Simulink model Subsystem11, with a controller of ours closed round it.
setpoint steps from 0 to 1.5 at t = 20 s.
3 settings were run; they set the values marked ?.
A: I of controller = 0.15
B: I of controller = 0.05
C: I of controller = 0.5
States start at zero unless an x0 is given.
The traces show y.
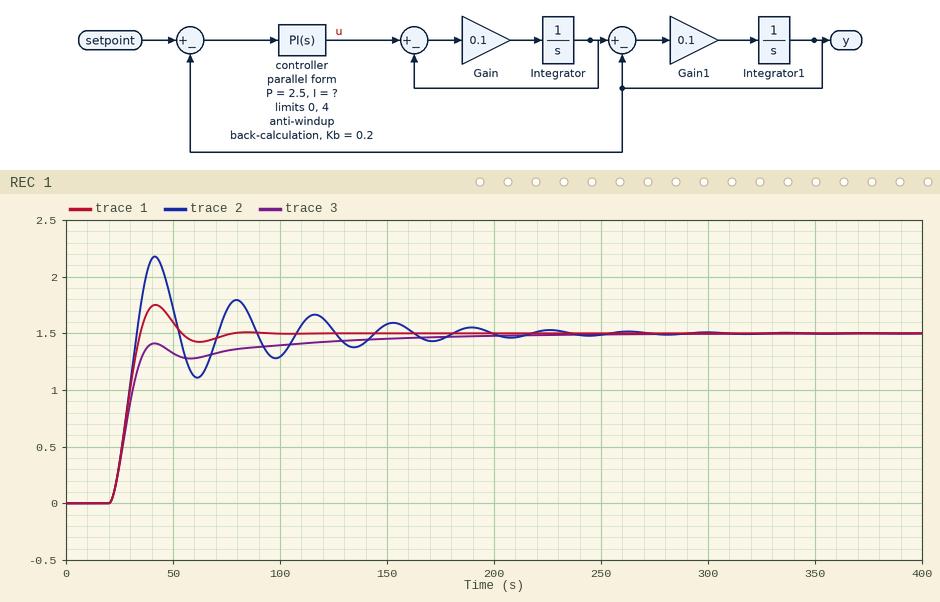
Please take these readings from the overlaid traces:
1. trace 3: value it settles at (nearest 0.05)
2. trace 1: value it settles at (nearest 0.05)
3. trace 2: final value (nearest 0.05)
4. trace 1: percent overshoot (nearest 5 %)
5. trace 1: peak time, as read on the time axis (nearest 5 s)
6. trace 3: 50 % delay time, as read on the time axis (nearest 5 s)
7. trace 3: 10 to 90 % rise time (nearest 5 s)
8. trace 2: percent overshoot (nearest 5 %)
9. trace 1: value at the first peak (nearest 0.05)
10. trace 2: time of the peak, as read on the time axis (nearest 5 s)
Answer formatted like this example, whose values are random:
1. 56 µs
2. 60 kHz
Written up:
1. 1.50
2. 1.50
3. 1.50
4. 15 %
5. 40 s
6. 30 s
7. 15 s
8. 45 %
9. 1.75
10. 40 s
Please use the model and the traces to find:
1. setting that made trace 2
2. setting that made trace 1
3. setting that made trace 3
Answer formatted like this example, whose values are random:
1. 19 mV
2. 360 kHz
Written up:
1. C
2. A
3. B
